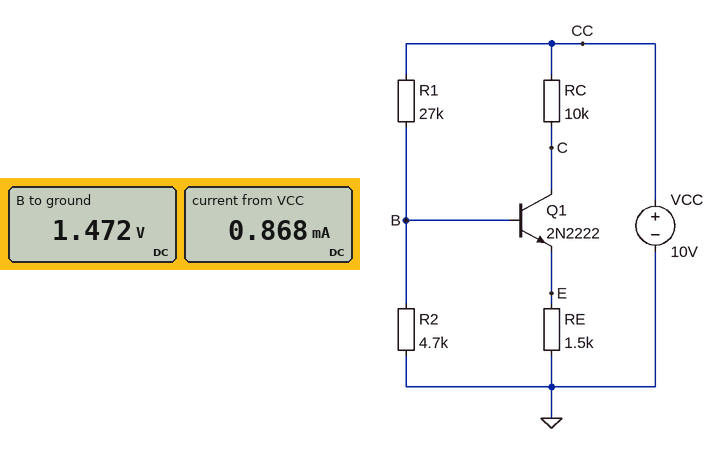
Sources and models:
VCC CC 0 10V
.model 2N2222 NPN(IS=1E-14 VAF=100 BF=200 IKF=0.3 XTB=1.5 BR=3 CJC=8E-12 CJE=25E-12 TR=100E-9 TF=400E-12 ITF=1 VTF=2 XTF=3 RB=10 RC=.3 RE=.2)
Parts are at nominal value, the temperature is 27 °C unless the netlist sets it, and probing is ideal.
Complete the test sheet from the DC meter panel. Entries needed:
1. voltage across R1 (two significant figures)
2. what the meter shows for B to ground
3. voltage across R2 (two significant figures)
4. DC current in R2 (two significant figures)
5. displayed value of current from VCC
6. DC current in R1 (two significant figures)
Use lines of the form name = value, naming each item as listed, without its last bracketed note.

voltage across R1 = 8.5 V
what the meter shows for B to ground = 1.472 V
voltage across R2 = 1.5 V
DC current in R2 = 310 µA
displayed value of current from VCC = 0.868 mA
DC current in R1 = 320 µA
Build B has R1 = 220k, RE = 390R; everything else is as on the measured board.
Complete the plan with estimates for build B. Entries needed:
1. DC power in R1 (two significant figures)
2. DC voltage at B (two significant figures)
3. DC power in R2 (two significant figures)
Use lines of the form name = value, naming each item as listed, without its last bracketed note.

DC power in R1 = 440 µW
DC voltage at B = 210 mV
DC power in R2 = 9.3 µW
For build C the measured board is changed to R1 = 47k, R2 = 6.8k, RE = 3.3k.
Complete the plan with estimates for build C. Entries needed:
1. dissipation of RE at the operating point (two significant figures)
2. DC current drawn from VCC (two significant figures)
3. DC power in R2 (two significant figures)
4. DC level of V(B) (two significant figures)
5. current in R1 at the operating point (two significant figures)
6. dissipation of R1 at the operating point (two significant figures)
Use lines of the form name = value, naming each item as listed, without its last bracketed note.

dissipation of RE at the operating point = 130 µW
DC current drawn from VCC = 380 µA
DC power in R2 = 230 µW
DC level of V(B) = 1.3 V
current in R1 at the operating point = 190 µA
dissipation of R1 at the operating point = 1.6 mW
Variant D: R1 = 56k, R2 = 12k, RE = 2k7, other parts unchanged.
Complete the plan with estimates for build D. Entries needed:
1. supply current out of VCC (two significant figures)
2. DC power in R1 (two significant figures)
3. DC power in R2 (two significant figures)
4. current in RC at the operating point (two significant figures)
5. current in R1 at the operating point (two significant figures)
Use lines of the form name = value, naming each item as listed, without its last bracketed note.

supply current out of VCC = 560 µA
DC power in R1 = 1.2 mW
DC power in R2 = 250 µW
current in RC at the operating point = 410 µA
current in R1 at the operating point = 150 µA
